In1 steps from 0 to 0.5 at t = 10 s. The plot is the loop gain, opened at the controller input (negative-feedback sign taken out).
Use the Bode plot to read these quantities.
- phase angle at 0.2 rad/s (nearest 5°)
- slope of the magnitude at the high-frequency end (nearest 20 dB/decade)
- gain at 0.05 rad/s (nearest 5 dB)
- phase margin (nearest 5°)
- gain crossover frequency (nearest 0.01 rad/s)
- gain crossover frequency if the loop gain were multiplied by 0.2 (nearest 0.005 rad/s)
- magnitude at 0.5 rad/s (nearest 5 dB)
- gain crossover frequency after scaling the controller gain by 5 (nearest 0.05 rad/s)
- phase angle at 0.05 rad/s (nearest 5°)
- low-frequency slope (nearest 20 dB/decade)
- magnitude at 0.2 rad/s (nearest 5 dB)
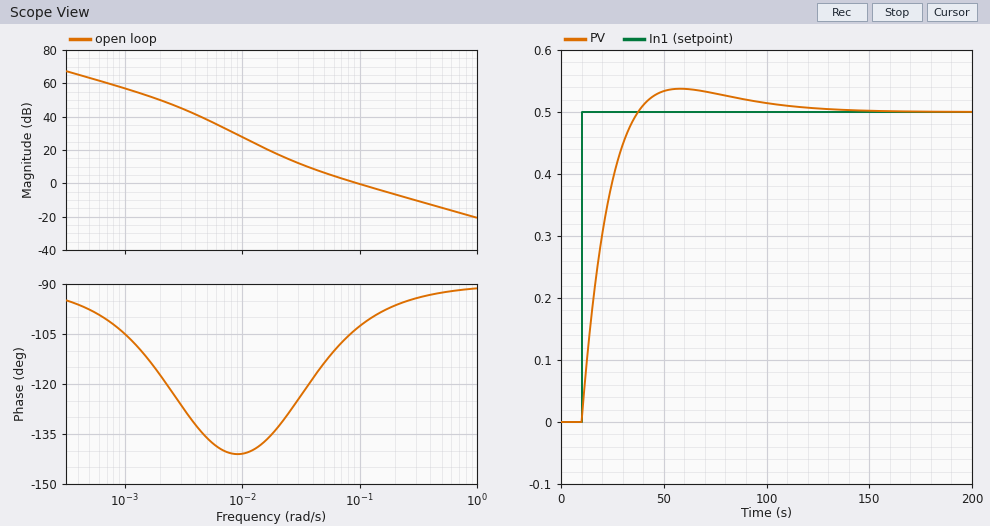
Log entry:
-95°
-20 dB/decade
5 dB
75°
0.10 rad/s
0.025 rad/s
-15 dB
0.45 rad/s
-115°
-20 dB/decade
-5 dB
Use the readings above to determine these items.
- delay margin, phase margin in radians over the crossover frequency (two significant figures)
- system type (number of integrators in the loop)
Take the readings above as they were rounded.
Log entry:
13 s
1
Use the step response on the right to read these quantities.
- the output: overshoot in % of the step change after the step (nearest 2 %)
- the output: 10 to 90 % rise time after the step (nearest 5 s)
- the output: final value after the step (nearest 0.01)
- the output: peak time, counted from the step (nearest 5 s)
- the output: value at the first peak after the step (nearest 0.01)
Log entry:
8 %
20 s
0.50
50 s
0.54
